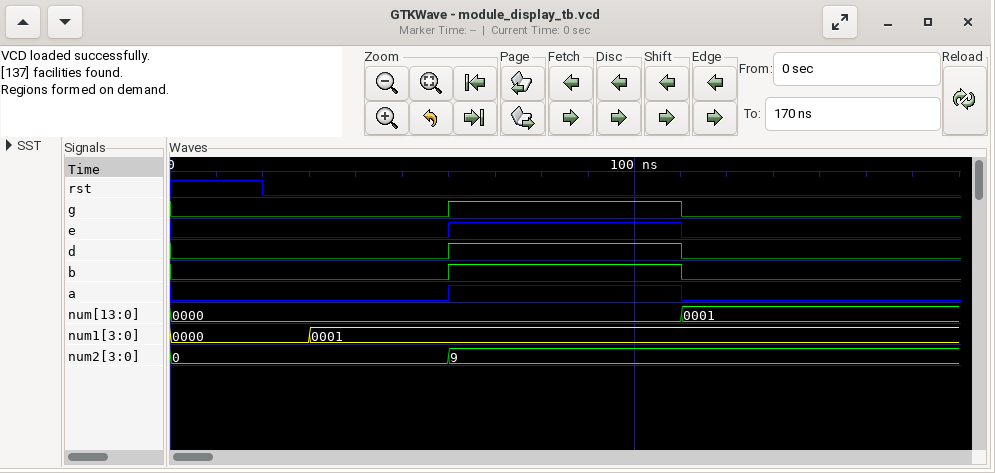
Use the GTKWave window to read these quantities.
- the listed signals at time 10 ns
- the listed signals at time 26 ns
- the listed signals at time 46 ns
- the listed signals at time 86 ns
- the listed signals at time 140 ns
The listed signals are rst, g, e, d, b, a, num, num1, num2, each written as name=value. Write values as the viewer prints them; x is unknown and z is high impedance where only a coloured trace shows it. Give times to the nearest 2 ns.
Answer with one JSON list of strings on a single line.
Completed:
["rst=1, g=0, e=0, d=0, b=0, a=0, num=0000, num1=0000, num2=0", "rst=0, g=0, e=0, d=0, b=0, a=0, num=0000, num1=0000, num2=0", "rst=0, g=0, e=0, d=0, b=0, a=0, num=0000, num1=0001, num2=0", "rst=0, g=1, e=1, d=1, b=1, a=1, num=0000, num1=0001, num2=9", "rst=0, g=0, e=0, d=0, b=0, a=0, num=0001, num1=0001, num2=9"]
